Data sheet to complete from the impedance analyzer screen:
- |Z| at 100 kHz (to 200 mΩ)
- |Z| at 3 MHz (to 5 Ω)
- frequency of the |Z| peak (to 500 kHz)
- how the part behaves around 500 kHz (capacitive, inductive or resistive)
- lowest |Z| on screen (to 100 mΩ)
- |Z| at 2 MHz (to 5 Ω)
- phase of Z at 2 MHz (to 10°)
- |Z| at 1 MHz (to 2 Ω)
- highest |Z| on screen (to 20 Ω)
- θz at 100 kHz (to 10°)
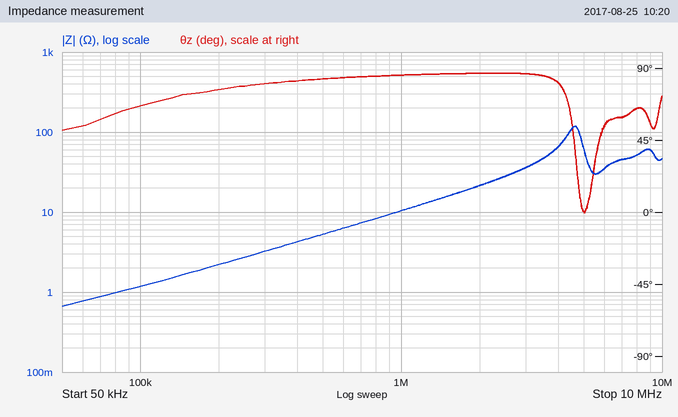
1.2 Ω
35 Ω
4.5 MHz
inductive
700 mΩ
20 Ω
90°
10 Ω
120 Ω
70°
